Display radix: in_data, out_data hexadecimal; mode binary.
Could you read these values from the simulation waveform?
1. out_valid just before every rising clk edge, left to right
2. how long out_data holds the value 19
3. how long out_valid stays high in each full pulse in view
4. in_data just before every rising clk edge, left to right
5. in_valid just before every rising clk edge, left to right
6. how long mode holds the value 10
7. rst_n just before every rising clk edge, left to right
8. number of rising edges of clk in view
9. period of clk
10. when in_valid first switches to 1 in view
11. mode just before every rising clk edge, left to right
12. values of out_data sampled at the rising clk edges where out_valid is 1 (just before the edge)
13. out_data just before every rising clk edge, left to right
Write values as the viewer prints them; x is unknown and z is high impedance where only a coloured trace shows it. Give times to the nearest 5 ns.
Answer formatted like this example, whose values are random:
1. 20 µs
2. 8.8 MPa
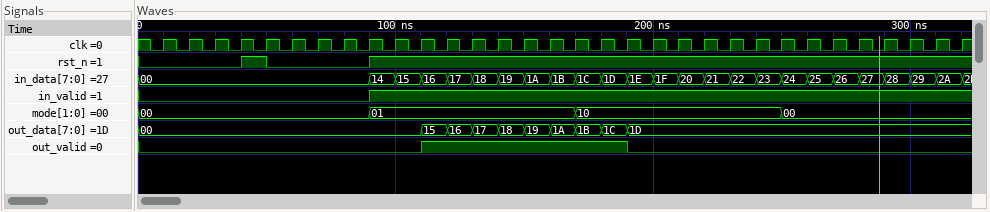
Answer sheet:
1. 0 0 0 0 0 0 0 0 0 0 0 1 1 1 1 1 1 1 1 0 0 0 0 0 0 0 0 0 0 0 0 0
2. 10 ns
3. 80 ns
4. 00, 00, 00, 00, 00, 00, 00, 00, 00, 14, 15, 16, 17, 18, 19, 1A, 1B, 1C, 1D, 1E, 1F, 20, 21, 22, 23, 24, 25, 26, 27, 28, 29, 2A
5. 0 0 0 0 0 0 0 0 0 1 1 1 1 1 1 1 1 1 1 1 1 1 1 1 1 1 1 1 1 1 1 1
6. 80 ns
7. 0 0 0 0 1 0 0 0 0 1 1 1 1 1 1 1 1 1 1 1 1 1 1 1 1 1 1 1 1 1 1 1
8. 32
9. 10 ns
10. 90 ns
11. 00, 00, 00, 00, 00, 00, 00, 00, 00, 01, 01, 01, 01, 01, 01, 01, 01, 10, 10, 10, 10, 10, 10, 10, 10, 00, 00, 00, 00, 00, 00, 00
12. 15, 16, 17, 18, 19, 1A, 1B, 1C
13. 00, 00, 00, 00, 00, 00, 00, 00, 00, 00, 00, 15, 16, 17, 18, 19, 1A, 1B, 1C, 1D, 1D, 1D, 1D, 1D, 1D, 1D, 1D, 1D, 1D, 1D, 1D, 1D
